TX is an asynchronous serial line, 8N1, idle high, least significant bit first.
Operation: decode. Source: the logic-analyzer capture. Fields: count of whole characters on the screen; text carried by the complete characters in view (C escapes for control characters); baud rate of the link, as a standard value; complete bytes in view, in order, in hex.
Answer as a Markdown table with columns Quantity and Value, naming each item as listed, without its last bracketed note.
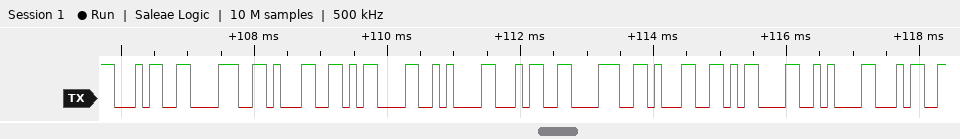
| Quantity | Value |
|---|---|
| count of whole characters on the screen | 11 |
| text carried by the complete characters in view | "481\r\n481\r\n4" |
| baud rate of the link, as a standard value | 9600 baud |
| complete bytes in view, in order, in hex | 34 38 31 0D 0A 34 38 31 0D 0A 34 |
